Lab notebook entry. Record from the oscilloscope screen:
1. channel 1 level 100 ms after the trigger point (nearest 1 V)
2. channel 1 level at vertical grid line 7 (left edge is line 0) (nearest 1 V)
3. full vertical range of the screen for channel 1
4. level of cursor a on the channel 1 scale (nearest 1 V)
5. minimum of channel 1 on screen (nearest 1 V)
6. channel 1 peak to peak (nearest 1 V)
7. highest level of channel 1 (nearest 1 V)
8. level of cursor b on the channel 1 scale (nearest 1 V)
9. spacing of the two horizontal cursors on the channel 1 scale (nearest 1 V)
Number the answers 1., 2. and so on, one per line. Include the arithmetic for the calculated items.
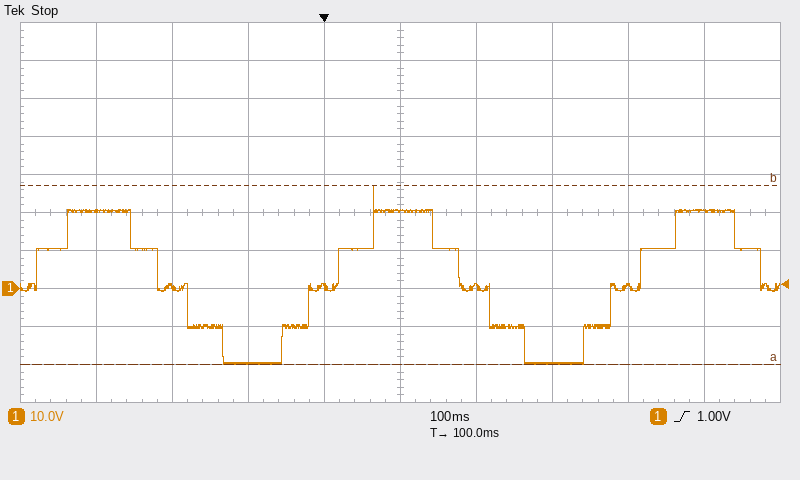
1. 20 V
2. -20 V
3. 100 V
4. -20 V
5. -20 V
6. 27 V − (-20 V) = 47 V
7. 27 V
8. 27 V
9. 47 V
